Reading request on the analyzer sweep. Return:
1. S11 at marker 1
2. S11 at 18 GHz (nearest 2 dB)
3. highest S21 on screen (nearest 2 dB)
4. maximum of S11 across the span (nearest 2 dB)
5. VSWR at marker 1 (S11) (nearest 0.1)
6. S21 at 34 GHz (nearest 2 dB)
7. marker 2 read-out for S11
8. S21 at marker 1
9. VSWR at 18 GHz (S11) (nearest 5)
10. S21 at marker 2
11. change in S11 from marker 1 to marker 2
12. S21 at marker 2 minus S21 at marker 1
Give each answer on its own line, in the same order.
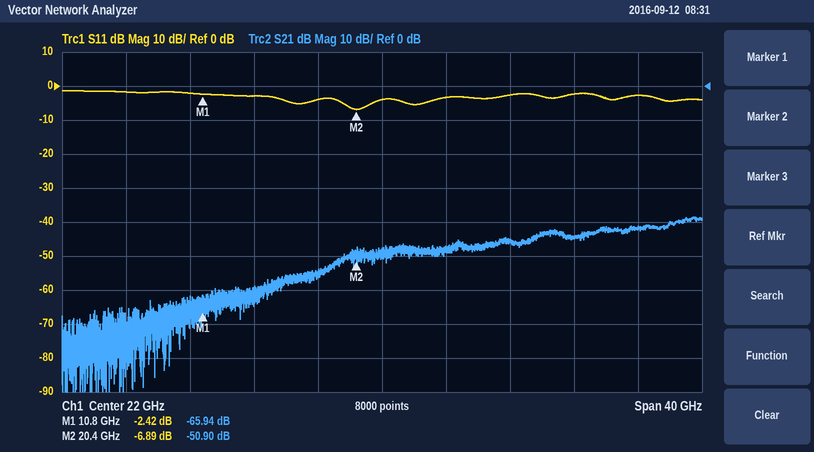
-2.42 dB
-4 dB
-38 dB
-2 dB
7.2
-44 dB
-6.89 dB
-65.94 dB
5
-50.90 dB
-4.47 dB
15.04 dB
